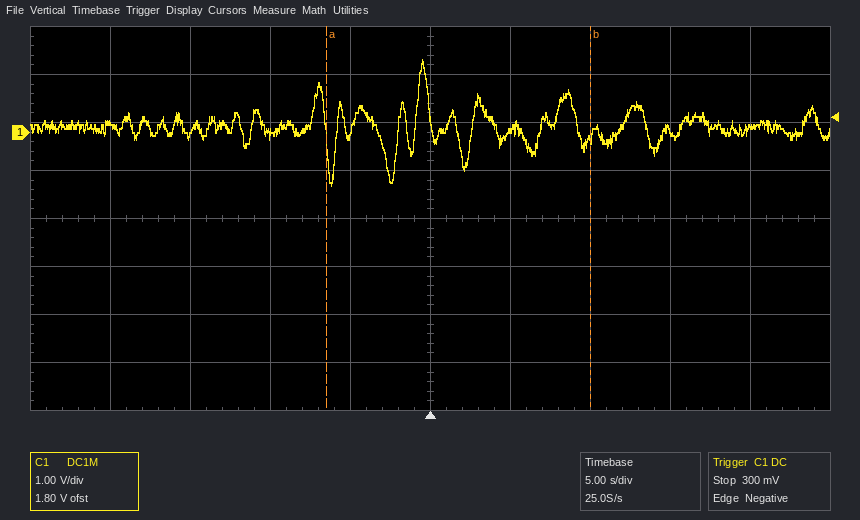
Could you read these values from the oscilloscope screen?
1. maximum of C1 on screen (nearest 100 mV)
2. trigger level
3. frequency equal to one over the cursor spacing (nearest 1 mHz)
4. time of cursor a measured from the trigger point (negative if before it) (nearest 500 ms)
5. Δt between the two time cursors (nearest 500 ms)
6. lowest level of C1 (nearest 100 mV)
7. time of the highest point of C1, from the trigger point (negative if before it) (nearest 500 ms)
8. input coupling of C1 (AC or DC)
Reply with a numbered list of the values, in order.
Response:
1. 1.5 V
2. 300 mV
3. 61 mHz
4. -6.5 s
5. 16.5 s
6. -1.1 V
7. -500 ms
8. DC
